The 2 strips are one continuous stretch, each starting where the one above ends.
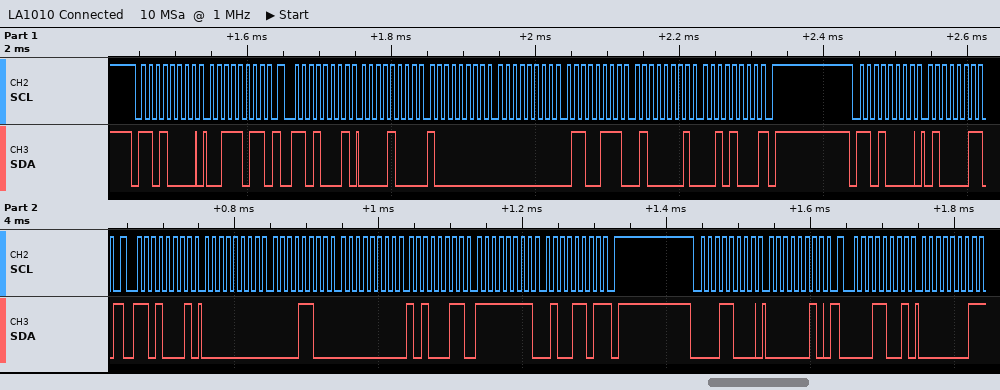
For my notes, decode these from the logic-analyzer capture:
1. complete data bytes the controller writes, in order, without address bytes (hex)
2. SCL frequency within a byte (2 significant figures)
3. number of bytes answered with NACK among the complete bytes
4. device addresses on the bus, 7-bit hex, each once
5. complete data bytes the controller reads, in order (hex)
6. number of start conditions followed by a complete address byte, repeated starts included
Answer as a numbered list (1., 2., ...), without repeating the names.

1. 3B 43 02
2. 100 kHz
3. 3
4. 0x68 0x0C
5. 08 80 00 67 41 28 00 0C 00 A3 FF 4D 01
6. 6
